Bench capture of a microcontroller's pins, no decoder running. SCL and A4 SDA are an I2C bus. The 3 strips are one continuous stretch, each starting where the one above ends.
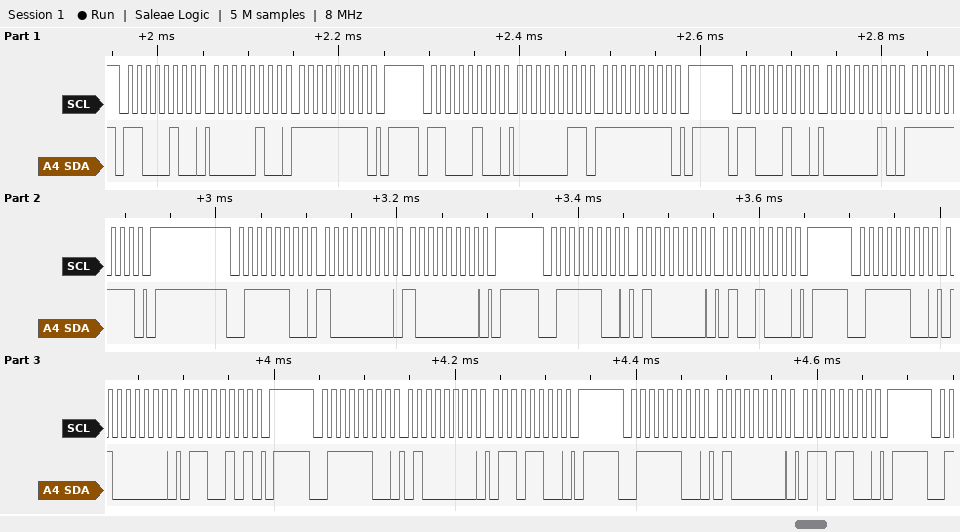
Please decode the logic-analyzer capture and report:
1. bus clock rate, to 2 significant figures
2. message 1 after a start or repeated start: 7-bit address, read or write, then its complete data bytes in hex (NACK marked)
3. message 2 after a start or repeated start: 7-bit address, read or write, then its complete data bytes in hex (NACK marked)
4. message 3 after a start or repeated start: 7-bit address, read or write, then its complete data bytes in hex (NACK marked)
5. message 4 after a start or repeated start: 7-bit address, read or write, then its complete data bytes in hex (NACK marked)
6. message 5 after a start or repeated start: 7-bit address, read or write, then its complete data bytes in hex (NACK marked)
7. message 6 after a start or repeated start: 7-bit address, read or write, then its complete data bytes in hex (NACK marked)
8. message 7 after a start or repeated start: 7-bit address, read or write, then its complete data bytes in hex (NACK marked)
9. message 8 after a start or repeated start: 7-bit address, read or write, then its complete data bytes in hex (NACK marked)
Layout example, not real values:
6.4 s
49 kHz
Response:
100 kHz
0x62 write: 04 FF
0x62 write: 03 FF
0x62 write: 02 FF
0x3E write: 80 80
0x3E write: 40 48
0x3E write: 40 65
0x3E write: 40 6C
0x3E write: 40 6C
